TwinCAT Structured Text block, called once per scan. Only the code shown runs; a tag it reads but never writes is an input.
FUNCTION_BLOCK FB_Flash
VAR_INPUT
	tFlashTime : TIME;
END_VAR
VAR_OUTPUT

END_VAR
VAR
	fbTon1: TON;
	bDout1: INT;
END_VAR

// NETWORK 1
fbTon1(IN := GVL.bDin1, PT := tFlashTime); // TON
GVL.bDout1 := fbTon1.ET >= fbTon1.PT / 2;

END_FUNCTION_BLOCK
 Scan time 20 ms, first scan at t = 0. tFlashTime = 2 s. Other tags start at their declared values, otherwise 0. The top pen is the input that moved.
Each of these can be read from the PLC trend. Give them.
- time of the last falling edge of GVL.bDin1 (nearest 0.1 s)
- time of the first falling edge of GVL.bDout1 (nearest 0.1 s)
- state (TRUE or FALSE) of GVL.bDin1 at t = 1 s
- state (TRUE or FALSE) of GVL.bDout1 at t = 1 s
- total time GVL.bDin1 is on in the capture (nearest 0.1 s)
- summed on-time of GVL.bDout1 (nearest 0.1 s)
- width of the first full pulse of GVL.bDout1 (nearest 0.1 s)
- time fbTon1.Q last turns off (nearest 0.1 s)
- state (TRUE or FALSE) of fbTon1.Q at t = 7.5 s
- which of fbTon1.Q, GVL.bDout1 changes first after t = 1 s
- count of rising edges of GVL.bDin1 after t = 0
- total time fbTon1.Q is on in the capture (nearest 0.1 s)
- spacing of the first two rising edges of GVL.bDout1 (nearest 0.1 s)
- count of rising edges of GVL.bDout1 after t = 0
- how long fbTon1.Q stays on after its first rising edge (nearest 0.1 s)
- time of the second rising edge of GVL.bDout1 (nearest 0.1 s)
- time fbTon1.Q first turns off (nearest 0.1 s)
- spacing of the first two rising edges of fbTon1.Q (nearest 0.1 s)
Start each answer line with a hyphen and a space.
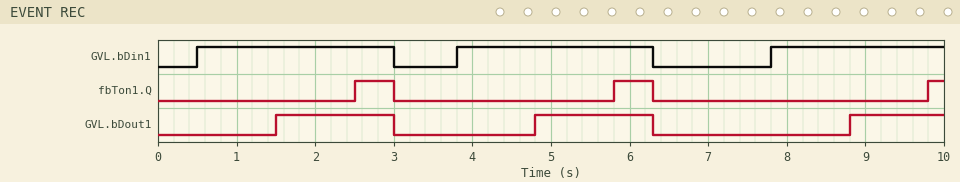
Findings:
- 6.3 s
- 3.0 s
- TRUE
- FALSE
- 7.2 s
- 4.2 s
- 1.5 s
- 6.3 s
- FALSE
- GVL.bDout1
- 3
- 1.2 s
- 3.3 s
- 3
- 0.5 s
- 4.8 s
- 3.0 s
- 3.3 s
